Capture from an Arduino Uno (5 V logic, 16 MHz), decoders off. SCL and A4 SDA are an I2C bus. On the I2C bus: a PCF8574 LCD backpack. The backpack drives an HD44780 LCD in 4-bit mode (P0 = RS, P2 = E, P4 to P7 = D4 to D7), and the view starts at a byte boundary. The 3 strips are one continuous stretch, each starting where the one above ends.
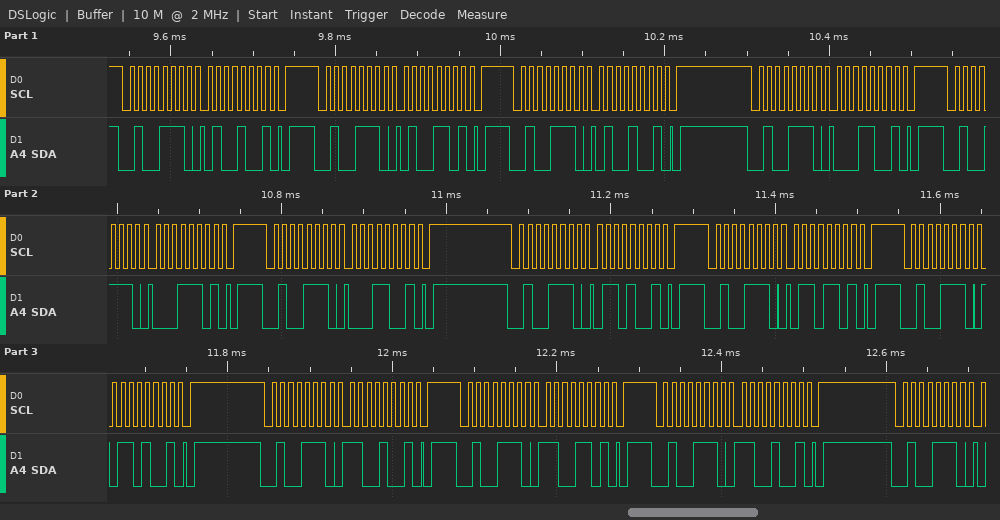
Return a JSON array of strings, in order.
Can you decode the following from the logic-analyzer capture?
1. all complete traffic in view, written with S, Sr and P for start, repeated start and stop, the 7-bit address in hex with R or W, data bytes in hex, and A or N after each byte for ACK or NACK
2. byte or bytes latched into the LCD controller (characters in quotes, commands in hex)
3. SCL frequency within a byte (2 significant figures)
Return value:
["S 27W A 49 A P S 27W A 4D A P S 27W A 49 A P S 27W A 19 A P S 27W A 1D A P S 27W A 19 A P S 27W A 69 A P S 27W A 6D A P S 27W A 69 A P S 27W A C9 A P S 27W A CD A P S 27W A C9 A P S 27W A", "'A' 'l'", "100 kHz"]
